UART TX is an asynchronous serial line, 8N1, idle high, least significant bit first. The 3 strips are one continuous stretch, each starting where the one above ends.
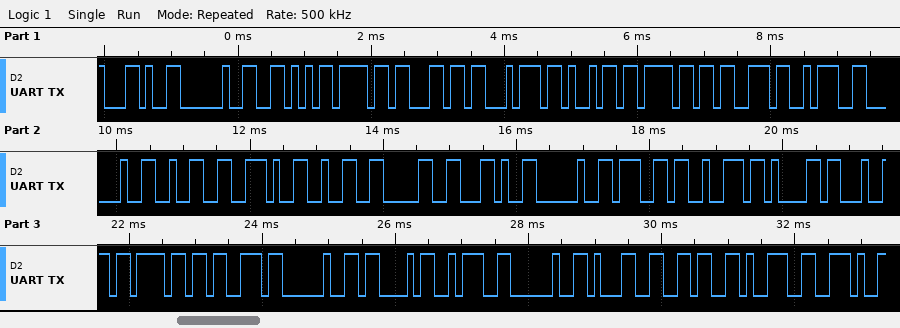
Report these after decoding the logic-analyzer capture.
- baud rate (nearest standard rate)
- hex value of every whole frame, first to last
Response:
9600 baud
0x2C 0x20 0x56 0x6F 0x6C 0x74 0x69 0x6F 0x73 0x3A 0x20 0x32 0x2E 0x32 0x30 0x2C 0x20 0x67 0x72 0x61 0x64 0x6F 0x73 0x20 0x43 0x3A 0x20 0x31 0x36 0x39 0x2E
